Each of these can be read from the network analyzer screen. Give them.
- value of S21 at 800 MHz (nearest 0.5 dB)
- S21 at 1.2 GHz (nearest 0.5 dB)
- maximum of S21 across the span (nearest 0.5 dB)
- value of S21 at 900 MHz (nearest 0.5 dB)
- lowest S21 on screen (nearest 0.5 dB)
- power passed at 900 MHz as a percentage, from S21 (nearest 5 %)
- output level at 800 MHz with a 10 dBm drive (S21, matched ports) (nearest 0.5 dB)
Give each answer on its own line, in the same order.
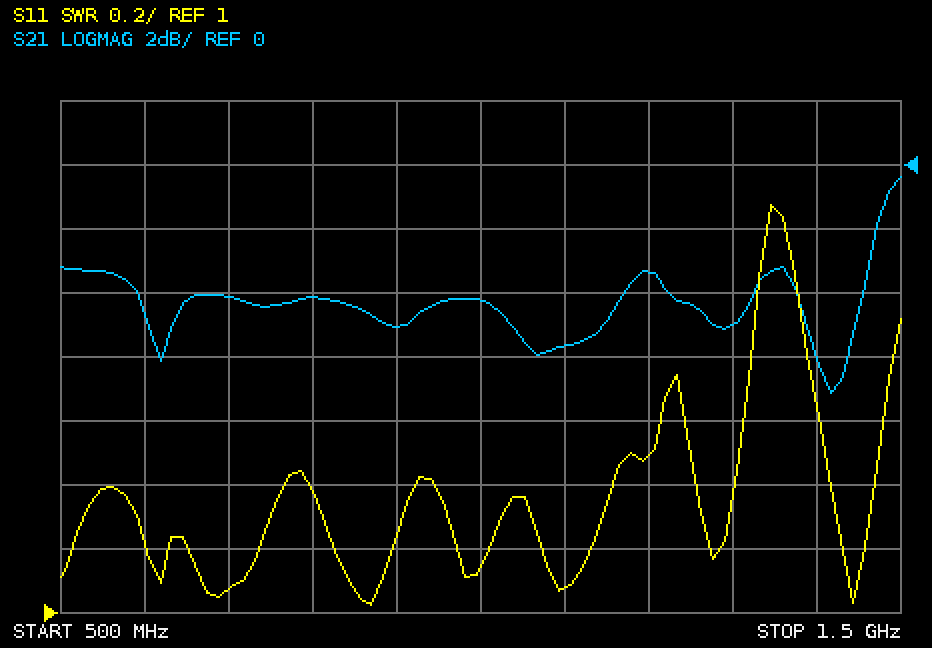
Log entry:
-4.0 dB
-3.5 dB
-0.5 dB
-5.0 dB
-7.0 dB
30 %
6.0 dBm
